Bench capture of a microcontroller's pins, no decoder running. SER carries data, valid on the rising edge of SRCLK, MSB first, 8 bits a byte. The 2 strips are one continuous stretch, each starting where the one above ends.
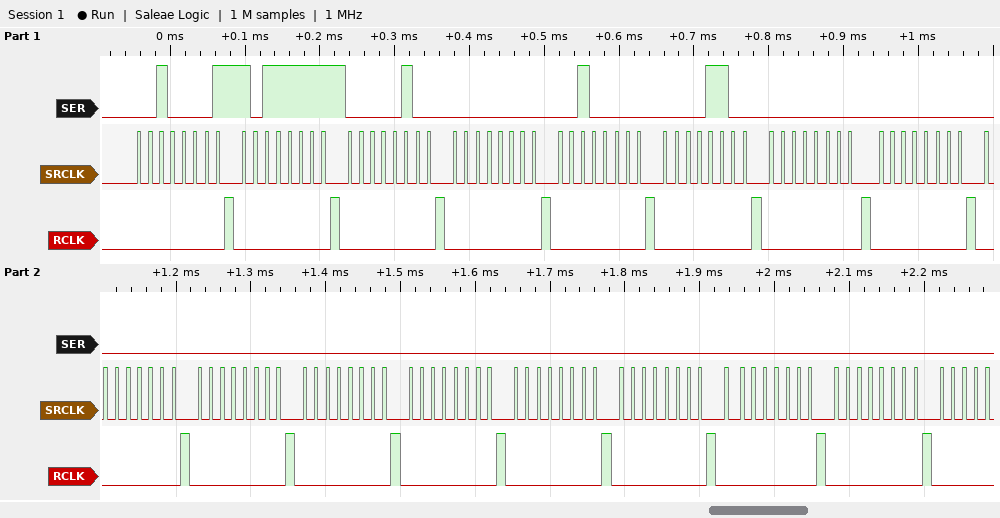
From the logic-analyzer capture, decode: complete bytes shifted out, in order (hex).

0x21 0xBF 0x04 0x00 0x20 0x0C 0x00 0x00 0x00 0x00 0x00 0x00 0x00 0x00 0x00 0x00
